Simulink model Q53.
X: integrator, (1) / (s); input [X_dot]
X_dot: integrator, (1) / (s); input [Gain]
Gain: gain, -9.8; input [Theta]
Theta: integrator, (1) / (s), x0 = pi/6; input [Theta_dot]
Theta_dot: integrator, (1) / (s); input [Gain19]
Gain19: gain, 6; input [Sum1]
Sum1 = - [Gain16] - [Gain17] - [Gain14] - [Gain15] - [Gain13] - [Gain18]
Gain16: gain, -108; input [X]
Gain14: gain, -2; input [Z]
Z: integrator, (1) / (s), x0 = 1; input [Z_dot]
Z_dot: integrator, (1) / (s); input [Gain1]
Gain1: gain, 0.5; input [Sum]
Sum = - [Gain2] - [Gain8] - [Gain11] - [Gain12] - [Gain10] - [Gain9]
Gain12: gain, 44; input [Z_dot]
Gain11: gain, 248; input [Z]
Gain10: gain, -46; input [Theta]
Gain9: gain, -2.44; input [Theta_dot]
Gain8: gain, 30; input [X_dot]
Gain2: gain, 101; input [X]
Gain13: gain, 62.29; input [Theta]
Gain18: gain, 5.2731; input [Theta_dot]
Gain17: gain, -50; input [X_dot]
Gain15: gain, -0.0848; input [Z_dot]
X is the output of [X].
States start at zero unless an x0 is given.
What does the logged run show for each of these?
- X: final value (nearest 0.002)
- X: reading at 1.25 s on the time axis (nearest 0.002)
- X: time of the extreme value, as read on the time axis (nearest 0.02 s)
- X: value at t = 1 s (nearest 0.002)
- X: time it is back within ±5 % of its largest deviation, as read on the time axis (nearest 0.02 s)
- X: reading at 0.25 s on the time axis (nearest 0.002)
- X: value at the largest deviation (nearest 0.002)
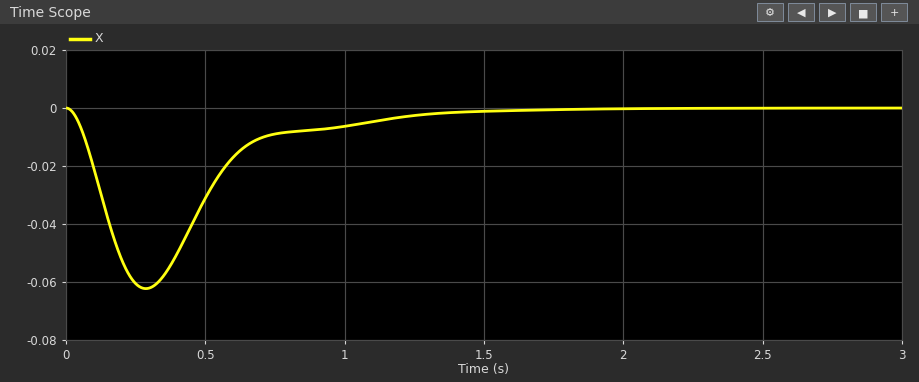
0.000
-0.002
0.28 s
-0.006
1.20 s
-0.060
-0.062
